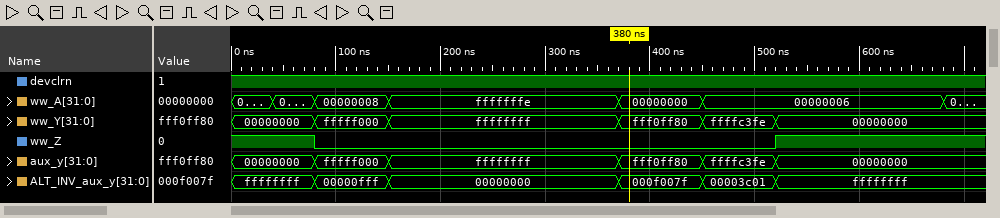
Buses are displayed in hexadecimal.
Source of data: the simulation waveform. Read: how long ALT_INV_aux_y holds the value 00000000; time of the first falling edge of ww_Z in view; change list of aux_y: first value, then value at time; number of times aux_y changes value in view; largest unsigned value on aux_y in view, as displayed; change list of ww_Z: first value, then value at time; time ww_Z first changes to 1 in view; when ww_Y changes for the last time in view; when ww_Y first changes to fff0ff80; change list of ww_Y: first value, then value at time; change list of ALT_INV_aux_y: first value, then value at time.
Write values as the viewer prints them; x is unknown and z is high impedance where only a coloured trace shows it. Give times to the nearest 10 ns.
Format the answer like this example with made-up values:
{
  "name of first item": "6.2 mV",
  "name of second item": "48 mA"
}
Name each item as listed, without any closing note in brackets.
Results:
{
  "how long ALT_INV_aux_y holds the value 00000000": "220 ns",
  "time of the first falling edge of ww_Z in view": "80 ns",
  "change list of aux_y: first value, then value at time": "00000000, fffff000 at 80 ns, ffffffff at 150 ns, fff0ff80 at 370 ns, ffffc3fe at 450 ns, 00000000 at 520 ns",
  "number of times aux_y changes value in view": "5",
  "largest unsigned value on aux_y in view, as displayed": "ffffffff",
  "change list of ww_Z: first value, then value at time": "1, 0 at 80 ns, 1 at 520 ns",
  "time ww_Z first changes to 1 in view": "520 ns",
  "when ww_Y changes for the last time in view": "520 ns",
  "when ww_Y first changes to fff0ff80": "370 ns",
  "change list of ww_Y: first value, then value at time": "00000000, fffff000 at 80 ns, ffffffff at 150 ns, fff0ff80 at 370 ns, ffffc3fe at 450 ns, 00000000 at 520 ns",
  "change list of ALT_INV_aux_y: first value, then value at time": "ffffffff, 00000fff at 80 ns, 00000000 at 150 ns, 000f007f at 370 ns, 00003c01 at 450 ns, ffffffff at 520 ns"
}
